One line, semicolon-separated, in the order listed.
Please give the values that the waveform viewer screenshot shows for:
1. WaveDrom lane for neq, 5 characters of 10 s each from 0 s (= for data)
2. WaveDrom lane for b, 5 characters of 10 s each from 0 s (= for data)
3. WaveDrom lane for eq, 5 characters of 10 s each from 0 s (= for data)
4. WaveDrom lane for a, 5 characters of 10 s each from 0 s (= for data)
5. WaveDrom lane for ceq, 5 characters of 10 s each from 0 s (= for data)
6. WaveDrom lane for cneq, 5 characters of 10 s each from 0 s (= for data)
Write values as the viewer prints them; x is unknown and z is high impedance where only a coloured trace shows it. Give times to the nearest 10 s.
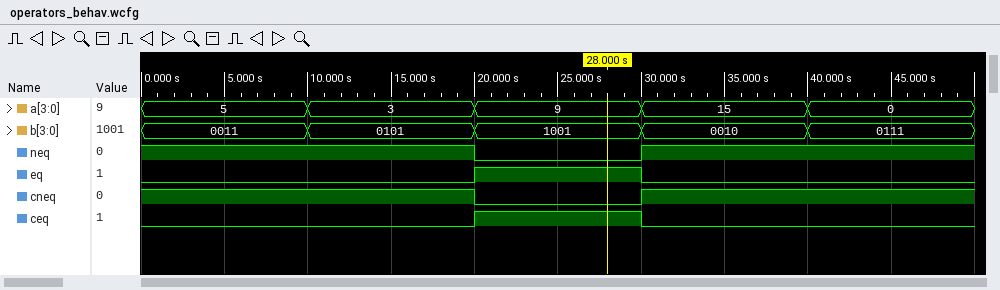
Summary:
{name: 'neq', wave: '1.01.'}; {name: 'b', wave: '=====', data: '0011 0101 1001 0010 0111'}; {name: 'eq', wave: '0.10.'}; {name: 'a', wave: '=====', data: '5 3 9 15 0'}; {name: 'ceq', wave: '0.10.'}; {name: 'cneq', wave: '1.01.'}
